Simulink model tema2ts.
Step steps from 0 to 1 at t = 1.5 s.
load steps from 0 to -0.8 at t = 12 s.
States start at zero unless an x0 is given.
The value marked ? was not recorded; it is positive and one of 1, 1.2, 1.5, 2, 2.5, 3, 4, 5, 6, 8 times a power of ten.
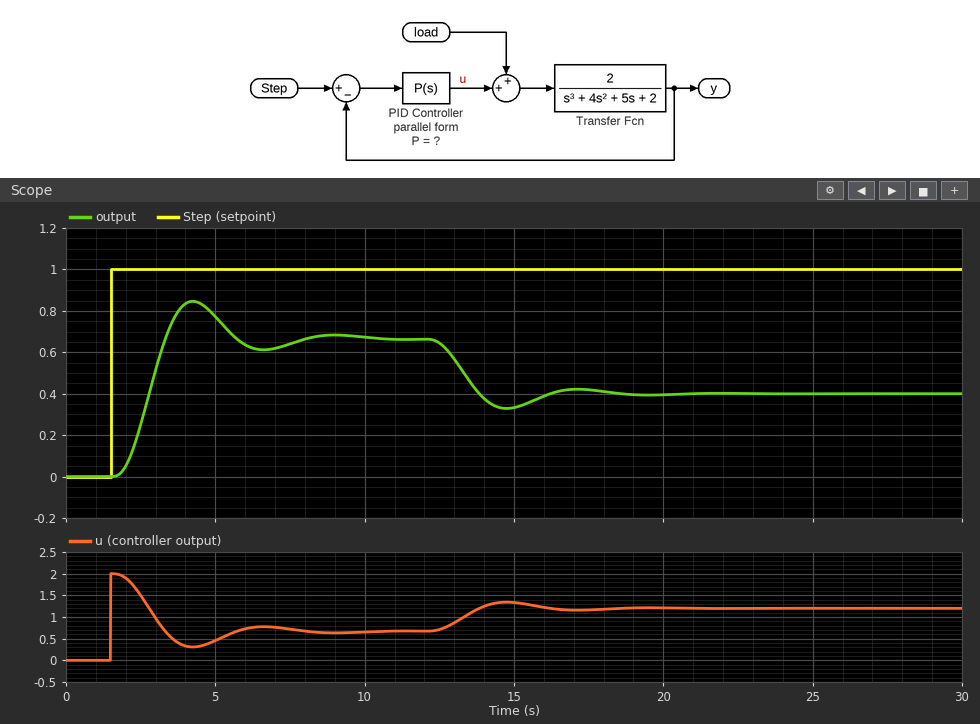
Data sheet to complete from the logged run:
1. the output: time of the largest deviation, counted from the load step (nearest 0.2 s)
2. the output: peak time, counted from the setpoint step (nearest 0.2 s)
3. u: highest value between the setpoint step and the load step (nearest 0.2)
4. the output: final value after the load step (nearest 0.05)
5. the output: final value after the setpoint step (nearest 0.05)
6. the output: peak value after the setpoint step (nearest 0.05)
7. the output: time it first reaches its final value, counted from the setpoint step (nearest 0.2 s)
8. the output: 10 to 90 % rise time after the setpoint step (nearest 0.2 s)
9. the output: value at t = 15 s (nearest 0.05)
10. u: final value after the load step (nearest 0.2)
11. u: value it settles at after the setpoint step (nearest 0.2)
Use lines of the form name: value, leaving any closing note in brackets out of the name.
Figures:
the output: time of the largest deviation, counted from the load step: 2.8 s
the output: peak time, counted from the setpoint step: 2.8 s
u: highest value between the setpoint step and the load step: 2.0
the output: final value after the load step: 0.40
the output: final value after the setpoint step: 0.65
the output: peak value after the setpoint step: 0.85
the output: time it first reaches its final value, counted from the setpoint step: 1.8 s
the output: 10 to 90 % rise time after the setpoint step: 1.2 s
the output: value at t = 15 s: 0.35
u: final value after the load step: 1.2
u: value it settles at after the setpoint step: 0.6
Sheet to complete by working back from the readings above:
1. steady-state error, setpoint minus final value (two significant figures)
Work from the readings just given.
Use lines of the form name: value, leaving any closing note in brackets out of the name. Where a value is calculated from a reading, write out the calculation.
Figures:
steady-state error, setpoint minus final value: 1 - 0.65 = 0.35
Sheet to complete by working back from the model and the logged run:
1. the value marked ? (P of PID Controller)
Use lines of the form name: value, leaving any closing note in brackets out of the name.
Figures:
the value marked ?: 2
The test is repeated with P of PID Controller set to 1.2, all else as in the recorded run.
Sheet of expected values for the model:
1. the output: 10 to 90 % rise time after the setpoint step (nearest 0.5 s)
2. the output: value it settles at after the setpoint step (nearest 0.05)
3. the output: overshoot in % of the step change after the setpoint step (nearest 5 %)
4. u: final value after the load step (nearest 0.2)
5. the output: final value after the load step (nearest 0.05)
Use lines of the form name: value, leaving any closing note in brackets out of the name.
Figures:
the output: 10 to 90 % rise time after the setpoint step: 1.5 s
the output: value it settles at after the setpoint step: 0.55
the output: overshoot in % of the step change after the setpoint step: 15 %
u: final value after the load step: 1.0
the output: final value after the load step: 0.20
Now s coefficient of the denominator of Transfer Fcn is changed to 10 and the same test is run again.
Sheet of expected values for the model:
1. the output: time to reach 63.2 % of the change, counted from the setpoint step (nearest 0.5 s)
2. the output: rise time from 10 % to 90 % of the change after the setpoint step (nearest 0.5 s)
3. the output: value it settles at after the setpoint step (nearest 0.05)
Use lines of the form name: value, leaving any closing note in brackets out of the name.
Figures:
the output: time to reach 63.2 % of the change, counted from the setpoint step: 1.5 s
the output: rise time from 10 % to 90 % of the change after the setpoint step: 2.5 s
the output: value it settles at after the setpoint step: 0.65
